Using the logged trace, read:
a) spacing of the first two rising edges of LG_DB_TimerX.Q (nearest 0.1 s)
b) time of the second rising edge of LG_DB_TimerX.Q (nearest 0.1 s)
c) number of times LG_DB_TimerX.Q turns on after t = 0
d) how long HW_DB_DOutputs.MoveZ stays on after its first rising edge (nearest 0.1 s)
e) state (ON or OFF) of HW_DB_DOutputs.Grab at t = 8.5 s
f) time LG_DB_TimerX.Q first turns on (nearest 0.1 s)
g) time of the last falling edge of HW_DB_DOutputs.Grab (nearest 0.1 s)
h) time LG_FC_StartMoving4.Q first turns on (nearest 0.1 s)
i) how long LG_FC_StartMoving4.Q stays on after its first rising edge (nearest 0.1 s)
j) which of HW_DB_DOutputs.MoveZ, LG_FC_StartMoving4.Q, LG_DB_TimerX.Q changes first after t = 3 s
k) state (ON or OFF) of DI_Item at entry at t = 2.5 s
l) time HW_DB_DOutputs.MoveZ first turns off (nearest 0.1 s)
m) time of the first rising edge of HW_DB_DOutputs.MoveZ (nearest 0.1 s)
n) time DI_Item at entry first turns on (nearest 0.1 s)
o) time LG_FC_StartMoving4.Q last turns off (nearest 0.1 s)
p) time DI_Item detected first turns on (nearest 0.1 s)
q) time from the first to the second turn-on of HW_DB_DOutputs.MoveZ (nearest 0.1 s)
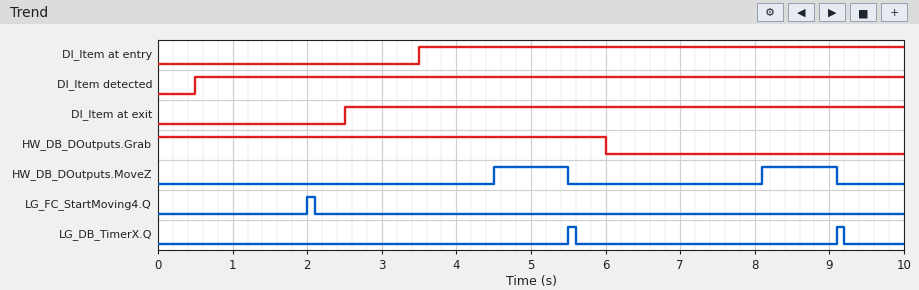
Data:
3.6 s
9.1 s
2
1.0 s
OFF
5.5 s
6.0 s
2.0 s
0.1 s
HW_DB_DOutputs.MoveZ
OFF
5.5 s
4.5 s
3.5 s
2.1 s
0.5 s
3.6 s
